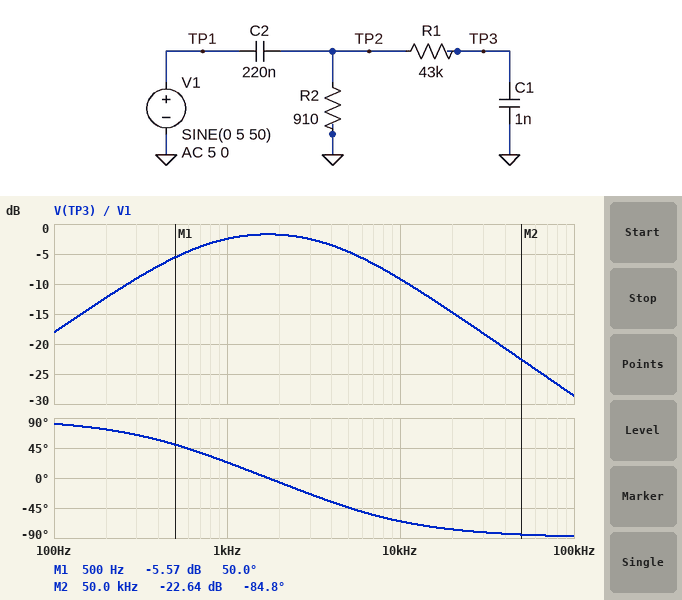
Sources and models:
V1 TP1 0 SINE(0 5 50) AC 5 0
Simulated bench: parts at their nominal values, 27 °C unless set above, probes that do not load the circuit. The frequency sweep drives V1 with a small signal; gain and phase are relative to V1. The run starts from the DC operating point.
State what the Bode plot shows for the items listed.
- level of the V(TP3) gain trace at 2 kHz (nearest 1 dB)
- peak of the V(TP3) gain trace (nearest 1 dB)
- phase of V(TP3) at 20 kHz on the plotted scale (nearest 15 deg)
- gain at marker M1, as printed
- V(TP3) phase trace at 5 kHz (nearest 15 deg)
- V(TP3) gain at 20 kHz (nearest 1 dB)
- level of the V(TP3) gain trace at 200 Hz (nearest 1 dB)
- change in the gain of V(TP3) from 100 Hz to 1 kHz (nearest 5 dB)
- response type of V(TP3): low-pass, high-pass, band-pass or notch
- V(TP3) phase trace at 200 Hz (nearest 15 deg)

-2 dB
-2 dB
-75 deg
-5.57 dB
-45 deg
-15 dB
-12 dB
15 dB
band-pass
75 deg
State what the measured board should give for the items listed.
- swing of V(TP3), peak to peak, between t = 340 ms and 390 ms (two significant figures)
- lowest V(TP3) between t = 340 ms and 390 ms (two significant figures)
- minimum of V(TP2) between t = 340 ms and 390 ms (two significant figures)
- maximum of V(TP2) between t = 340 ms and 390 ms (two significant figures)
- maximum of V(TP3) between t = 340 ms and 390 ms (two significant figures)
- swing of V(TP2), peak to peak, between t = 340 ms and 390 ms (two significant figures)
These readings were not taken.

630 mV
-310 mV
-310 mV
310 mV
310 mV
630 mV
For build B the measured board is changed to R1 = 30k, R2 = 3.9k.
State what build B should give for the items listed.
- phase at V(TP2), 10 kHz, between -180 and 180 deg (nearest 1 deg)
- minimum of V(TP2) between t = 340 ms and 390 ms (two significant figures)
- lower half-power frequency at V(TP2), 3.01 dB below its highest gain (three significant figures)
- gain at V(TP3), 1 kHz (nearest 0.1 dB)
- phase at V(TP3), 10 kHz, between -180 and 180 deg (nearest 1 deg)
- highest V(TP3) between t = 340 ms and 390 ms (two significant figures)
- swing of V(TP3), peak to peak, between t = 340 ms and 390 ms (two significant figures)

1 deg
-1.3 V
186 Hz
-0.3 dB
-61 deg
1.3 V
2.6 V
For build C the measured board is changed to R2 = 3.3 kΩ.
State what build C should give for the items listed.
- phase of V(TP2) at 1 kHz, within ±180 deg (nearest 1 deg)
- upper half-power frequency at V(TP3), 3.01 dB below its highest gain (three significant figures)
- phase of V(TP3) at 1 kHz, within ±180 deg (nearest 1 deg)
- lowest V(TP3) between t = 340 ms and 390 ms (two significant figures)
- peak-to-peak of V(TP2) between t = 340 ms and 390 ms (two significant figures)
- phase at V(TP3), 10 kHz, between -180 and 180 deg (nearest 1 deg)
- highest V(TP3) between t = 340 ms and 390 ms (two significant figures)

12 deg
4.13 kHz
-3 deg
-1.1 V
2.2 V
-68 deg
1.1 V
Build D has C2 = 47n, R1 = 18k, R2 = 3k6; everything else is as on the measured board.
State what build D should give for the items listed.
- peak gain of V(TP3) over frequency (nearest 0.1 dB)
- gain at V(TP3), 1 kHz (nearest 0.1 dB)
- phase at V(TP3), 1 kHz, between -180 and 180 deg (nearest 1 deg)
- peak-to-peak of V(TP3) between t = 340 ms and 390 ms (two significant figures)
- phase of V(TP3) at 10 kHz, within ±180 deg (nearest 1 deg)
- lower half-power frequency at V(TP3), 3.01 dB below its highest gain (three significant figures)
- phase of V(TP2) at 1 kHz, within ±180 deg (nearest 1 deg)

-1.0 dB
-2.9 dB
36 deg
530 mV
-43 deg
774 Hz
43 deg
